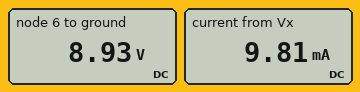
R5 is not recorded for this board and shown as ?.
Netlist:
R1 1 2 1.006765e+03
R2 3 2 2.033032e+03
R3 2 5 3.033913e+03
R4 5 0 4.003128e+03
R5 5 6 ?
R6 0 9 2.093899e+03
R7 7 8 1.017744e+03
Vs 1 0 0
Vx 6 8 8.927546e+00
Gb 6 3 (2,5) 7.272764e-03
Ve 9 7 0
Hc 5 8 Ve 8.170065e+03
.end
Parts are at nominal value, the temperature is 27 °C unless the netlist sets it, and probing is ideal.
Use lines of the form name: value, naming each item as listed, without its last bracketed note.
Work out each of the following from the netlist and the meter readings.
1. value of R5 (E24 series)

value of R5: 910 Ω
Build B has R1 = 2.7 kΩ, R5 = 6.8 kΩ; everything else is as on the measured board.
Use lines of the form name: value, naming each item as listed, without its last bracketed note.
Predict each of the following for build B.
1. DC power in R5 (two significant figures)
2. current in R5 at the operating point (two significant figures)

DC power in R5: 12 mW
current in R5 at the operating point: 1.3 mA
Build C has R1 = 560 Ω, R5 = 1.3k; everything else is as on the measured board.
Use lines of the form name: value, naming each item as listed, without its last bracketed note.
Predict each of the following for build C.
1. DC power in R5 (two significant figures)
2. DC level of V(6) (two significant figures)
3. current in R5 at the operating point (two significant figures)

DC power in R5: 61 mW
DC level of V(6): 8.9 V
current in R5 at the operating point: 6.9 mA
